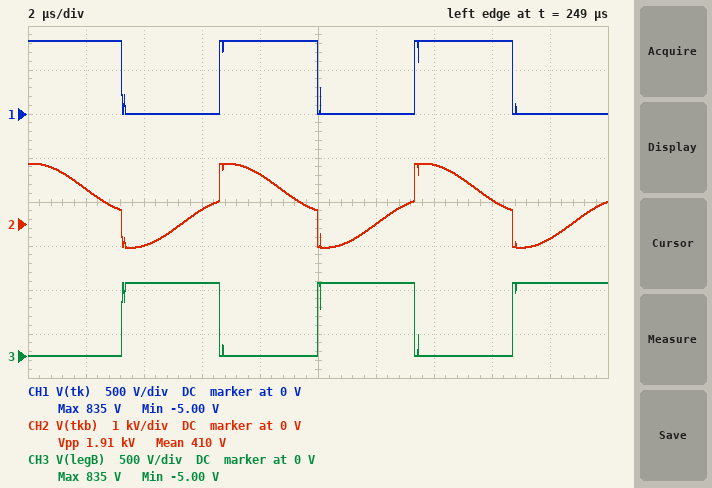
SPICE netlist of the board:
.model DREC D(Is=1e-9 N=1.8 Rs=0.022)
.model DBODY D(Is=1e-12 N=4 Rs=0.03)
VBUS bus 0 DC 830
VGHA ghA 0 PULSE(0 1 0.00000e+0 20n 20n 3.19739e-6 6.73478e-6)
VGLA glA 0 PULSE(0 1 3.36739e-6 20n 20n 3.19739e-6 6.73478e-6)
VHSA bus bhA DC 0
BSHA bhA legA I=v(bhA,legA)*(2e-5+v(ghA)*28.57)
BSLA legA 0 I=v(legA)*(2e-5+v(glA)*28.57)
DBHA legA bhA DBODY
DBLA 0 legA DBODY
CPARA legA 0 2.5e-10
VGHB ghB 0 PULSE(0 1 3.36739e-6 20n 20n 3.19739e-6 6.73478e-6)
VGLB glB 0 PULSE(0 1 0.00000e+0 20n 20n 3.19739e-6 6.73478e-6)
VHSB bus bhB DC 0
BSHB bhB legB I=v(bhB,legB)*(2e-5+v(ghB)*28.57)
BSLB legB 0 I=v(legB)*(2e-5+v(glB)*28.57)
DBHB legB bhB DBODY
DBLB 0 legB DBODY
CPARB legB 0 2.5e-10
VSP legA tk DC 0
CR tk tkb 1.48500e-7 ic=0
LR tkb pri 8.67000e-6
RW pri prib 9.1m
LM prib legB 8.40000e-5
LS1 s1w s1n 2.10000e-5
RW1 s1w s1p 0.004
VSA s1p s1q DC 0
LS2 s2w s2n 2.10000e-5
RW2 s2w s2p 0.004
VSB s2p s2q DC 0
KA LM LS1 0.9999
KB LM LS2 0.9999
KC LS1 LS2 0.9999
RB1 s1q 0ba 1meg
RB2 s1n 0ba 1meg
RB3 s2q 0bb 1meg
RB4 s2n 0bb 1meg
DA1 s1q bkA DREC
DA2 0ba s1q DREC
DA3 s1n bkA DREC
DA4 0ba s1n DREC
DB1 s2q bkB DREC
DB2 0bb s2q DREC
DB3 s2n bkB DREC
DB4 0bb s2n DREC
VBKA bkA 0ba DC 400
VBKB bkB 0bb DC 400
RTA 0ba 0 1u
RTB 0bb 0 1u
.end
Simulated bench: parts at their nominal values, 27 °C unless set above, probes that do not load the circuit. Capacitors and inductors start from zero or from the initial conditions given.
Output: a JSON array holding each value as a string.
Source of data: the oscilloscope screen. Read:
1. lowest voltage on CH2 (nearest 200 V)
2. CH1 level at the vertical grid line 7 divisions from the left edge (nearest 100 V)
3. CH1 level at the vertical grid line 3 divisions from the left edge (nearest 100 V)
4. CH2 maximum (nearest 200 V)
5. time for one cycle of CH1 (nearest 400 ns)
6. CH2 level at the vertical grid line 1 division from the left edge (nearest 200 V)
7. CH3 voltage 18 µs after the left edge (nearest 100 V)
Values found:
["-600 V", "800 V", "0 V", "1.4 kV", "6.8 µs", "800 V", "800 V"]
